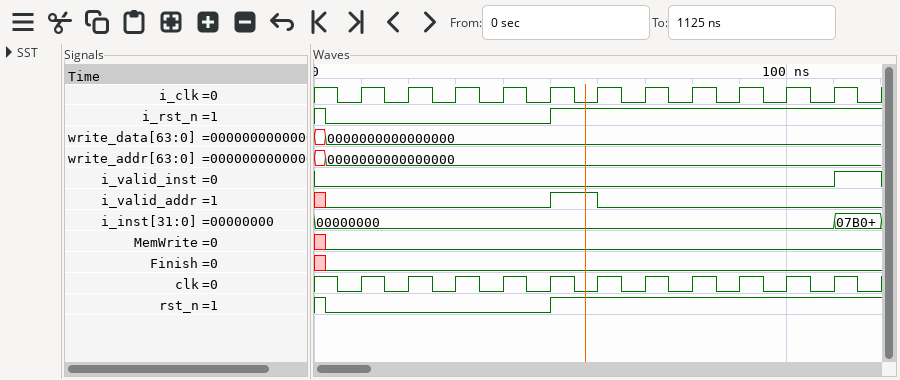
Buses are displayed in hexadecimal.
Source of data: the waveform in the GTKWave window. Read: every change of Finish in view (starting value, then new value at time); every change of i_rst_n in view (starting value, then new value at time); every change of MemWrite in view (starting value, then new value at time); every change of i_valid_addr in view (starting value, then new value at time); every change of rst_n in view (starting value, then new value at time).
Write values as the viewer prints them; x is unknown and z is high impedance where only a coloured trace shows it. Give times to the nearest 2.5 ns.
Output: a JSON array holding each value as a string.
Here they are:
["x, 0 at 2.5 ns", "1, 0 at 2.5 ns, 1 at 50 ns", "x, 0 at 2.5 ns", "x, 0 at 2.5 ns, 1 at 50 ns, 0 at 60 ns", "1, 0 at 2.5 ns, 1 at 50 ns"]
